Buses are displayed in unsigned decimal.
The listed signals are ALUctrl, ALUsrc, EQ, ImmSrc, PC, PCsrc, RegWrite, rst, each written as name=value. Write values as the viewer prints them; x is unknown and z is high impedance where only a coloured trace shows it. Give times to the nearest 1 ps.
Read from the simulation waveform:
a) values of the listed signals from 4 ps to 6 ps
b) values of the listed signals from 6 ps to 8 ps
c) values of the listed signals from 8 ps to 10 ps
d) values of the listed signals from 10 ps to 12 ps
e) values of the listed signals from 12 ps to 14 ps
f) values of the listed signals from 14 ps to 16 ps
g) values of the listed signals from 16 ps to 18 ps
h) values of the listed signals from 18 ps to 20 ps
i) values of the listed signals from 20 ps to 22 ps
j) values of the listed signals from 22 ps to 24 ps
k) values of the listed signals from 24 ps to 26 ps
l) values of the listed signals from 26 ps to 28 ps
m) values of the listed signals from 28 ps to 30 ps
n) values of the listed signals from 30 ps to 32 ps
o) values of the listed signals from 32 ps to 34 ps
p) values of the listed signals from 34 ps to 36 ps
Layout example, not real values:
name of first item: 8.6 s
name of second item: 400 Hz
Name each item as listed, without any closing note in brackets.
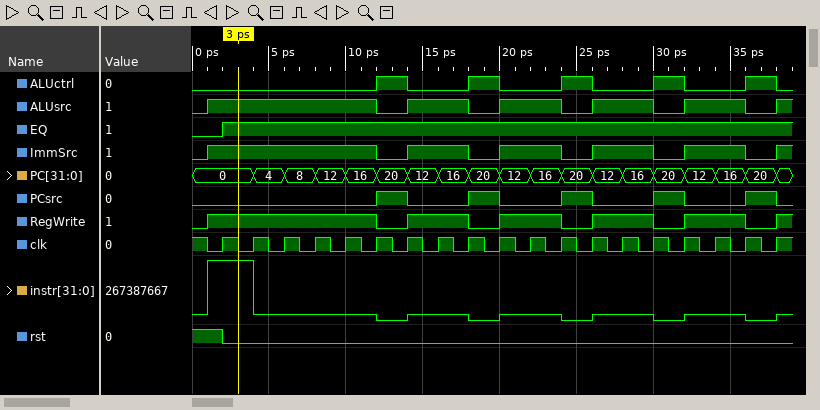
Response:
values of the listed signals from 4 ps to 6 ps: ALUctrl=0, ALUsrc=1, EQ=1, ImmSrc=1, PC=4, PCsrc=0, RegWrite=1, rst=0
values of the listed signals from 6 ps to 8 ps: ALUctrl=0, ALUsrc=1, EQ=1, ImmSrc=1, PC=8, PCsrc=0, RegWrite=1, rst=0
values of the listed signals from 8 ps to 10 ps: ALUctrl=0, ALUsrc=1, EQ=1, ImmSrc=1, PC=12, PCsrc=0, RegWrite=1, rst=0
values of the listed signals from 10 ps to 12 ps: ALUctrl=0, ALUsrc=1, EQ=1, ImmSrc=1, PC=16, PCsrc=0, RegWrite=1, rst=0
values of the listed signals from 12 ps to 14 ps: ALUctrl=1, ALUsrc=0, EQ=1, ImmSrc=0, PC=20, PCsrc=1, RegWrite=0, rst=0
values of the listed signals from 14 ps to 16 ps: ALUctrl=0, ALUsrc=1, EQ=1, ImmSrc=1, PC=12, PCsrc=0, RegWrite=1, rst=0
values of the listed signals from 16 ps to 18 ps: ALUctrl=0, ALUsrc=1, EQ=1, ImmSrc=1, PC=16, PCsrc=0, RegWrite=1, rst=0
values of the listed signals from 18 ps to 20 ps: ALUctrl=1, ALUsrc=0, EQ=1, ImmSrc=0, PC=20, PCsrc=1, RegWrite=0, rst=0
values of the listed signals from 20 ps to 22 ps: ALUctrl=0, ALUsrc=1, EQ=1, ImmSrc=1, PC=12, PCsrc=0, RegWrite=1, rst=0
values of the listed signals from 22 ps to 24 ps: ALUctrl=0, ALUsrc=1, EQ=1, ImmSrc=1, PC=16, PCsrc=0, RegWrite=1, rst=0
values of the listed signals from 24 ps to 26 ps: ALUctrl=1, ALUsrc=0, EQ=1, ImmSrc=0, PC=20, PCsrc=1, RegWrite=0, rst=0
values of the listed signals from 26 ps to 28 ps: ALUctrl=0, ALUsrc=1, EQ=1, ImmSrc=1, PC=12, PCsrc=0, RegWrite=1, rst=0
values of the listed signals from 28 ps to 30 ps: ALUctrl=0, ALUsrc=1, EQ=1, ImmSrc=1, PC=16, PCsrc=0, RegWrite=1, rst=0
values of the listed signals from 30 ps to 32 ps: ALUctrl=1, ALUsrc=0, EQ=1, ImmSrc=0, PC=20, PCsrc=1, RegWrite=0, rst=0
values of the listed signals from 32 ps to 34 ps: ALUctrl=0, ALUsrc=1, EQ=1, ImmSrc=1, PC=12, PCsrc=0, RegWrite=1, rst=0
values of the listed signals from 34 ps to 36 ps: ALUctrl=0, ALUsrc=1, EQ=1, ImmSrc=1, PC=16, PCsrc=0, RegWrite=1, rst=0
